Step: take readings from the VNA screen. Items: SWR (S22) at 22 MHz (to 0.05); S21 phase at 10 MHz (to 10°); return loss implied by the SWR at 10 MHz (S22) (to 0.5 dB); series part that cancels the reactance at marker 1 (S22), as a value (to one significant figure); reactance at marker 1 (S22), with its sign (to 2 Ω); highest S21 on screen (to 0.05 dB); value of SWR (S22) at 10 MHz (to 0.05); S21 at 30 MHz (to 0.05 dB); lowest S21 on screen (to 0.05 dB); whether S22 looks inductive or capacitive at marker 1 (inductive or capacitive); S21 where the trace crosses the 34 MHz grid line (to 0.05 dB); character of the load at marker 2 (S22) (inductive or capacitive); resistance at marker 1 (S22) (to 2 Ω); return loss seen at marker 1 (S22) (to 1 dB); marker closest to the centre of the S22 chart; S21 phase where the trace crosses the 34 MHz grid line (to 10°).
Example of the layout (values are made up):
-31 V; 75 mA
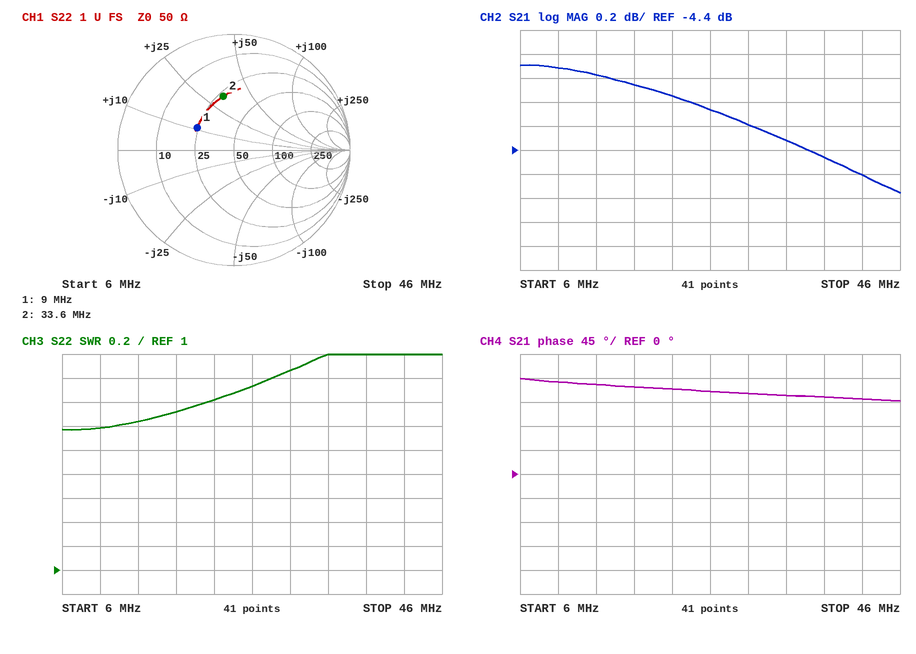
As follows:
2.40; 170°; 8.5 dB; 2 nF; +10 Ω; -3.70 dB; 2.20; -4.20 dB; -4.75 dB; inductive; -4.30 dB; inductive; 24 Ω; 9 dB; marker 1; 150°
